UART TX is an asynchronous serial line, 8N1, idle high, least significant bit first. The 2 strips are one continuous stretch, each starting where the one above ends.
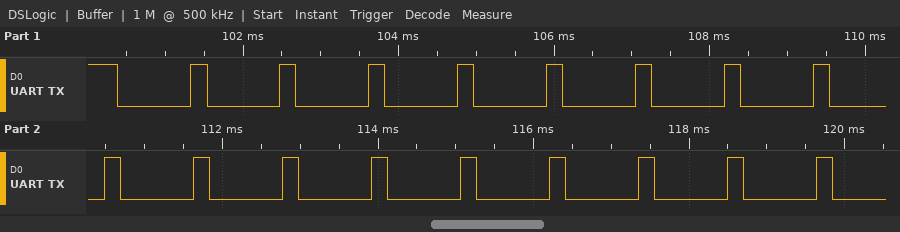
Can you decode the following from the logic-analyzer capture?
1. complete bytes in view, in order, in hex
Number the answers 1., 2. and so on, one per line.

1. 0x00 0x00 0x00 0x00 0x00 0x00 0x00 0x00 0x00 0x00 0x00 0x00 0x00 0x00 0x00 0x00 0x00
